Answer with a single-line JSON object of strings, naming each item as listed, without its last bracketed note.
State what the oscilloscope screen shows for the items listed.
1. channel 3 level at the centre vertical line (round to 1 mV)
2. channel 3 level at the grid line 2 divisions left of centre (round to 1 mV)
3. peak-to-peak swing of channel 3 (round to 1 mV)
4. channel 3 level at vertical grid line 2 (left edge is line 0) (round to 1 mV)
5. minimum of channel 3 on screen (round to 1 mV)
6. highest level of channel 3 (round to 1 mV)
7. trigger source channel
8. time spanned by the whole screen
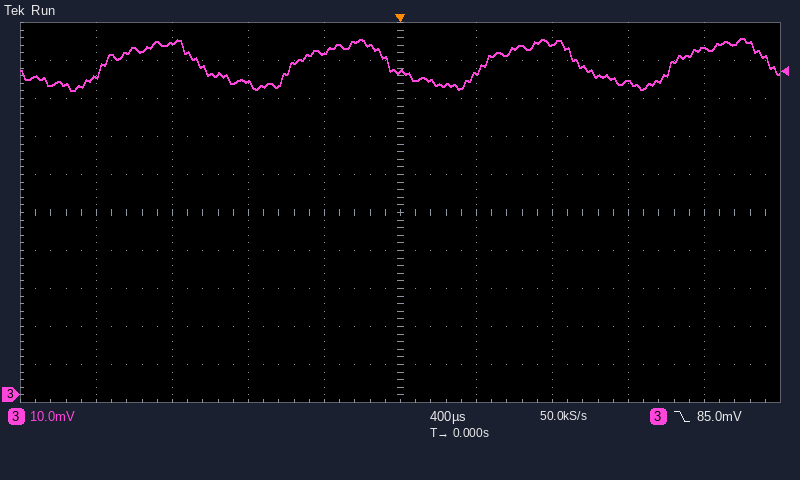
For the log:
{"channel 3 level at the centre vertical line": "85 mV", "channel 3 level at the grid line 2 divisions left of centre": "82 mV", "peak-to-peak swing of channel 3": "14 mV", "channel 3 level at vertical grid line 2 (left edge is line 0)": "93 mV", "minimum of channel 3 on screen": "80 mV", "highest level of channel 3": "94 mV", "trigger source channel": "channel 3", "time spanned by the whole screen": "4 ms"}
